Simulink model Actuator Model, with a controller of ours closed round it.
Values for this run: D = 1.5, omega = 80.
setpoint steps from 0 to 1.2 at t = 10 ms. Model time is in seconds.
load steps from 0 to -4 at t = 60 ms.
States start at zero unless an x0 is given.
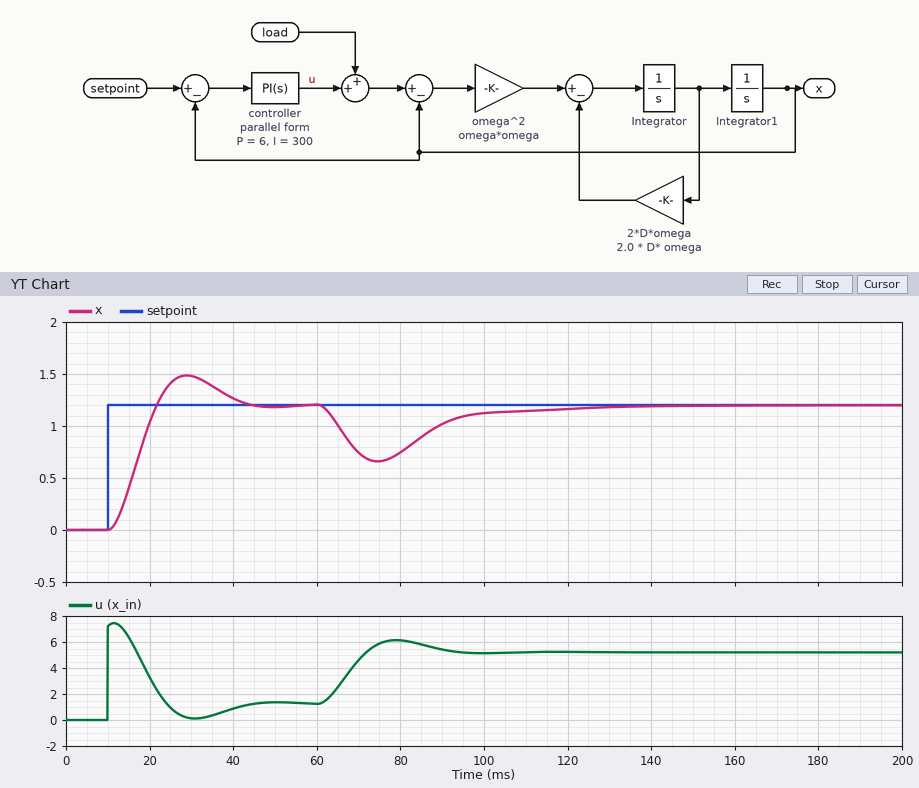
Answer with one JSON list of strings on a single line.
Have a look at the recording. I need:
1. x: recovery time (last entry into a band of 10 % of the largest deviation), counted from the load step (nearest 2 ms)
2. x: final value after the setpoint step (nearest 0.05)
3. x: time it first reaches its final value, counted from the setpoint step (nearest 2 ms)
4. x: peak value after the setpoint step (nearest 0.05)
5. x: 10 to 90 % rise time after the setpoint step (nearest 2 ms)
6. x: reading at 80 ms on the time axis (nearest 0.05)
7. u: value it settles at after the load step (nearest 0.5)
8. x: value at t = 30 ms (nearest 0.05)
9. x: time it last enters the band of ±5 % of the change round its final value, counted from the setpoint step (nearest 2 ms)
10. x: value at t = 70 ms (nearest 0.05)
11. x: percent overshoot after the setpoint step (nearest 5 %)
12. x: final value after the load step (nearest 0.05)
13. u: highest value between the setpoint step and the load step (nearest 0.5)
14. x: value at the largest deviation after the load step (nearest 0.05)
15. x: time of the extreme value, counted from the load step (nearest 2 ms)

["52 ms", "1.20", "12 ms", "1.50", "8 ms", "0.75", "5.0", "1.50", "30 ms", "0.75", "25 %", "1.20", "7.5", "0.65", "14 ms"]
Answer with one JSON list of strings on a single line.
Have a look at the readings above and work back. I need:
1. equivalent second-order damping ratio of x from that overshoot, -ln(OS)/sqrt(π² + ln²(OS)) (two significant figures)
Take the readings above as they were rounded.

["0.40"]
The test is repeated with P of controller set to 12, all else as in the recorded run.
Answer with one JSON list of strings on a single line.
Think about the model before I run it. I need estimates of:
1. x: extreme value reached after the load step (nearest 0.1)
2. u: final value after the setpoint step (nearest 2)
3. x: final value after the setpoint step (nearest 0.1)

["0.8", "2", "1.2"]
